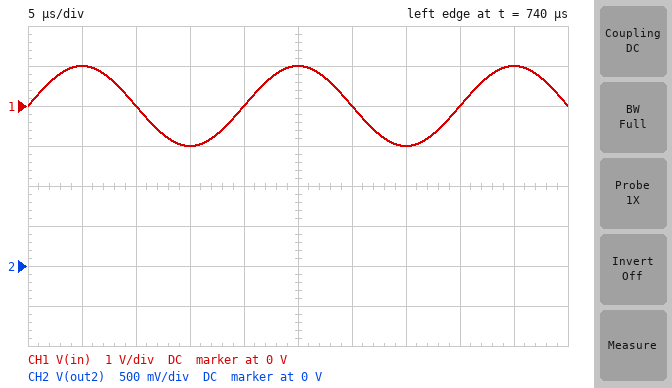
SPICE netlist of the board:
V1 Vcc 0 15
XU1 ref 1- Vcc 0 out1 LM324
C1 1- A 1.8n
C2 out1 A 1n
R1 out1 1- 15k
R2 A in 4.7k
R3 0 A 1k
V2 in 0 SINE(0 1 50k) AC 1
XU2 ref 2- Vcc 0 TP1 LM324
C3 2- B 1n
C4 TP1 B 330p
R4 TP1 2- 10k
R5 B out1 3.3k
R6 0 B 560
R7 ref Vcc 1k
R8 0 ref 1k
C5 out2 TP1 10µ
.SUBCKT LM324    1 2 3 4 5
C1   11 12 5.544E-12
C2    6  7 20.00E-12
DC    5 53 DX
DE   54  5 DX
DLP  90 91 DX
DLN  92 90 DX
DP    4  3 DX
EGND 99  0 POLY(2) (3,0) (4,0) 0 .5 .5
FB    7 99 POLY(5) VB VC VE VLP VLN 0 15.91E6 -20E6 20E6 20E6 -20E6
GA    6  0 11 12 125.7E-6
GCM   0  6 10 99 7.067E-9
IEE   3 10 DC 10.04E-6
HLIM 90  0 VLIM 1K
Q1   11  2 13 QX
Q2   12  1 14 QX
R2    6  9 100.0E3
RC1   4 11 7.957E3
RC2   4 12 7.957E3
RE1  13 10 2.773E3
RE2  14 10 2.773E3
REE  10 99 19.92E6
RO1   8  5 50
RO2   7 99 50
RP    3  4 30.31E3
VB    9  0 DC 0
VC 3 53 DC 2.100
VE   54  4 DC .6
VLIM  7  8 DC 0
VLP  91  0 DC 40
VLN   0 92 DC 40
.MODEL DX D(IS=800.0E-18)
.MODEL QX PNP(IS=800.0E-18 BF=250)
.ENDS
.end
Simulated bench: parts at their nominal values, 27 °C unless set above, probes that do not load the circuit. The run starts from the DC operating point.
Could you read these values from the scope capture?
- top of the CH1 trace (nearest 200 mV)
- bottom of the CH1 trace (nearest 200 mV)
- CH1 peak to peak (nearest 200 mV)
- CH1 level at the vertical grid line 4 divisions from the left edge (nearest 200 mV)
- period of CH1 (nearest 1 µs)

1.0 V
-1.0 V
2.0 V
0 V
20 µs
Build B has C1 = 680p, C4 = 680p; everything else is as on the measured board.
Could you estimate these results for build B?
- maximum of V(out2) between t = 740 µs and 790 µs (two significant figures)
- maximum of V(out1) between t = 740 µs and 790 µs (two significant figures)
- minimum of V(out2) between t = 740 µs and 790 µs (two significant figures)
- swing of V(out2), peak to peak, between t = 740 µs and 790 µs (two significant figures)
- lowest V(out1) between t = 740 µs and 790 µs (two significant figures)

8.5 V
8.8 V
6.5 V
2.1 V
6.2 V
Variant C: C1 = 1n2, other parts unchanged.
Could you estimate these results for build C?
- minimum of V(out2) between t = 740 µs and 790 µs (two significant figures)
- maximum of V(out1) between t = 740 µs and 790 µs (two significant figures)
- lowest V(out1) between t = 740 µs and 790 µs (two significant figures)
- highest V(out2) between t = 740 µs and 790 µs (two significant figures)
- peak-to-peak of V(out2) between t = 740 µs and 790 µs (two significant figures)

6.8 V
8.5 V
6.5 V
8.2 V
1.3 V
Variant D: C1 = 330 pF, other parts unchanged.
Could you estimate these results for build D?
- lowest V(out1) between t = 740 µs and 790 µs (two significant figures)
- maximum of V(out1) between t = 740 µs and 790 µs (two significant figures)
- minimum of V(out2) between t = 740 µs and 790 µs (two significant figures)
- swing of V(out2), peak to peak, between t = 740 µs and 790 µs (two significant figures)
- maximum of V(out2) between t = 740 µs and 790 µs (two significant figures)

7.1 V
7.9 V
7.2 V
560 mV
7.8 V
